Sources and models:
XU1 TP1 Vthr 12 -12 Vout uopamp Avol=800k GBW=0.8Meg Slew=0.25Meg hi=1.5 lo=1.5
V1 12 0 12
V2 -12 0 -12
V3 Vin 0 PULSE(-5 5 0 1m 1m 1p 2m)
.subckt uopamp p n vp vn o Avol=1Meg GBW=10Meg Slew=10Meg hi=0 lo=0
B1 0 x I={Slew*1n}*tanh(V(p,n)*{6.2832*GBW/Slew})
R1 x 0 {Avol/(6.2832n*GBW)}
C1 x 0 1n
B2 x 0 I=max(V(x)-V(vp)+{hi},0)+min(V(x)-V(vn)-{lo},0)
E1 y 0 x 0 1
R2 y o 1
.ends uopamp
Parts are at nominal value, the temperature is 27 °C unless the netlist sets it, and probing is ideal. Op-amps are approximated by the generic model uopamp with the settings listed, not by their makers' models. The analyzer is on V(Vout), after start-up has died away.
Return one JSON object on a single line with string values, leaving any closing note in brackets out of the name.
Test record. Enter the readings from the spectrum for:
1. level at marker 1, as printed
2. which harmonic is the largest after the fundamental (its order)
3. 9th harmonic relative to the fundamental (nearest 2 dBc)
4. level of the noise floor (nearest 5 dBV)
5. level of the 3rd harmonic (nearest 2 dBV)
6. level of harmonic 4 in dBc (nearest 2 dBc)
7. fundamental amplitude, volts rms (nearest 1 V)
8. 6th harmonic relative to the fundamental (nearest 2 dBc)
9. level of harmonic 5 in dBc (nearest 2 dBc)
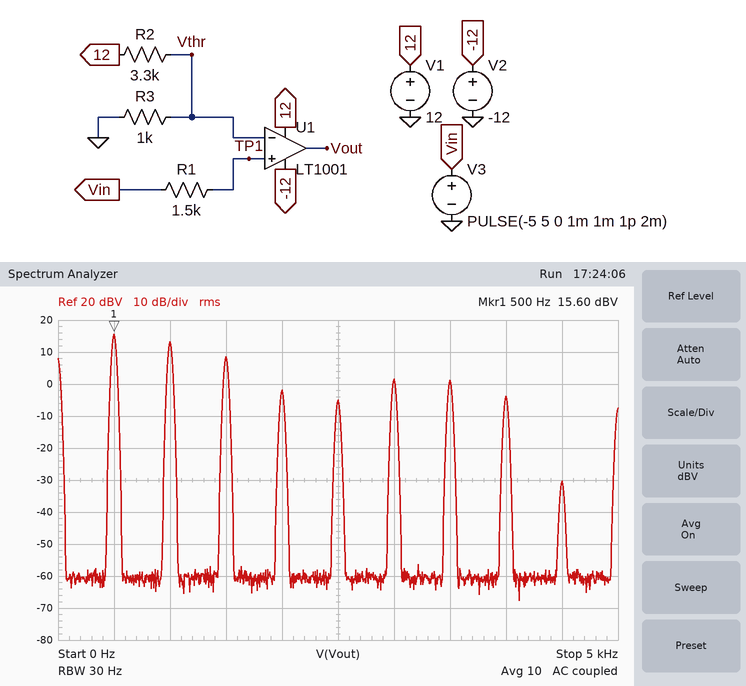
{"level at marker 1, as printed": "15.60 dBV", "which harmonic is the largest after the fundamental": "2", "9th harmonic relative to the fundamental": "-46 dBc", "level of the noise floor": "-60 dBV", "level of the 3rd harmonic": "8 dBV", "level of harmonic 4 in dBc": "-18 dBc", "fundamental amplitude, volts rms": "6 V", "6th harmonic relative to the fundamental": "-14 dBc", "level of harmonic 5 in dBc": "-20 dBc"}
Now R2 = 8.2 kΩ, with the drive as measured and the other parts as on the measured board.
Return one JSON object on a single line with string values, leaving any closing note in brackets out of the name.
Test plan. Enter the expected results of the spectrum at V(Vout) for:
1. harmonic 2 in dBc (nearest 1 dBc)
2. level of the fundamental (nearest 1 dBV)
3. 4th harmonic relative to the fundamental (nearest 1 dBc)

{"harmonic 2 in dBc": "-8 dBc", "level of the fundamental": "19 dBV", "4th harmonic relative to the fundamental": "-12 dBc"}
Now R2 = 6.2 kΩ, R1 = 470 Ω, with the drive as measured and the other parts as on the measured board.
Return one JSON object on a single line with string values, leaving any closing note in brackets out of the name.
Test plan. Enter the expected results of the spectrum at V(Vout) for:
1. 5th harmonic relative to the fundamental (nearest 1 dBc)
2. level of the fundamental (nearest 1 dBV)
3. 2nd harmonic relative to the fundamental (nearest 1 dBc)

{"5th harmonic relative to the fundamental": "-15 dBc", "level of the fundamental": "18 dBV", "2nd harmonic relative to the fundamental": "-6 dBc"}
